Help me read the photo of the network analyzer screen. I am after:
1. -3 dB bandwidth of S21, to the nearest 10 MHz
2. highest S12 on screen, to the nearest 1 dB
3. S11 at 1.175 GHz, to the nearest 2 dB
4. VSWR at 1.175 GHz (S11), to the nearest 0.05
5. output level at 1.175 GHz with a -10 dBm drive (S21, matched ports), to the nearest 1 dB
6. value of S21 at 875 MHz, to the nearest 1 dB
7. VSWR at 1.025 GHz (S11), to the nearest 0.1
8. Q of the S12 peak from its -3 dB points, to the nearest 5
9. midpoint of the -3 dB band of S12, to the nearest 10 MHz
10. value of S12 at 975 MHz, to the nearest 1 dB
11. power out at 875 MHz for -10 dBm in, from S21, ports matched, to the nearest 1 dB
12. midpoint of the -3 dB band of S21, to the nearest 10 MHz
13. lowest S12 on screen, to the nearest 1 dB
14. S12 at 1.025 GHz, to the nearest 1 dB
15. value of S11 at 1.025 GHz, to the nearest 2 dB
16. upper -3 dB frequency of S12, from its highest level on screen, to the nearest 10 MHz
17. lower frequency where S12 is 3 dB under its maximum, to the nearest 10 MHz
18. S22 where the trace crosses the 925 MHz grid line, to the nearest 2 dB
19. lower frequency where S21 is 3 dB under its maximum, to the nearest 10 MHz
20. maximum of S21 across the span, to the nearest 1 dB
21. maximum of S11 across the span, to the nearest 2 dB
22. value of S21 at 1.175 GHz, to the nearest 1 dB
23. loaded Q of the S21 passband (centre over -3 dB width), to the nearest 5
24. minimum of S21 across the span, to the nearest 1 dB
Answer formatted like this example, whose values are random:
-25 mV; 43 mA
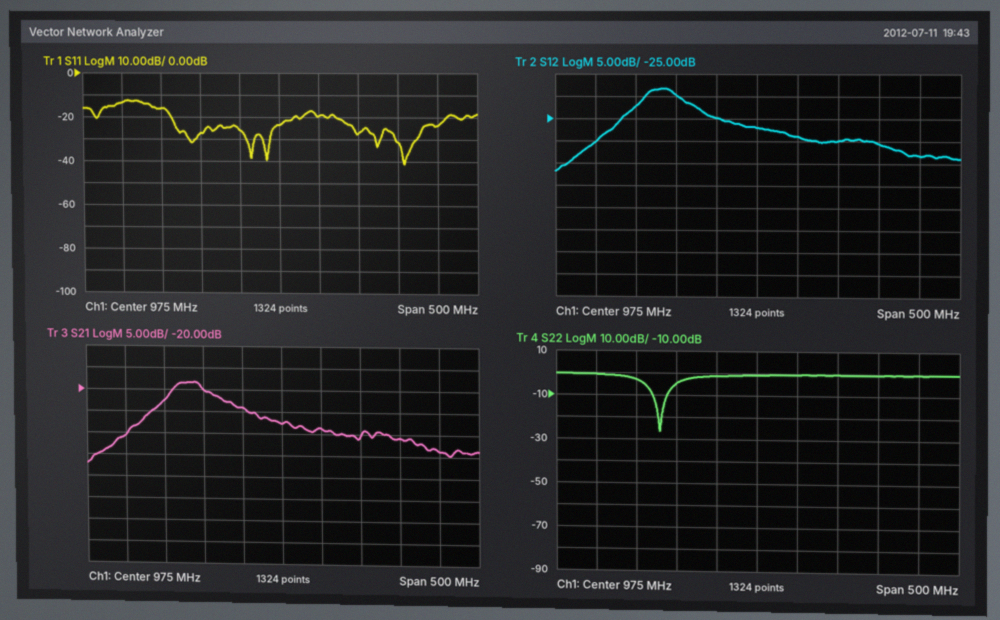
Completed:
60 MHz; -18 dB; -24 dB; 1.15; -44 dBm; -20 dB; 1.2; 15; 860 MHz; -27 dB; -30 dBm; 860 MHz; -37 dB; -29 dB; -20 dB; 890 MHz; 830 MHz; -2 dB; 830 MHz; -18 dB; -12 dB; -34 dB; 15; -37 dB
